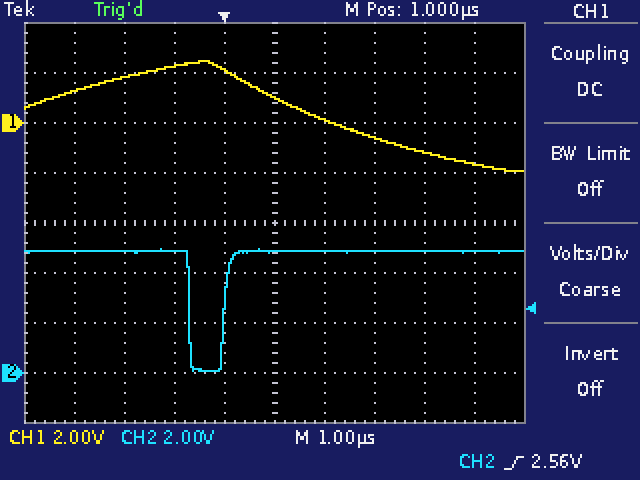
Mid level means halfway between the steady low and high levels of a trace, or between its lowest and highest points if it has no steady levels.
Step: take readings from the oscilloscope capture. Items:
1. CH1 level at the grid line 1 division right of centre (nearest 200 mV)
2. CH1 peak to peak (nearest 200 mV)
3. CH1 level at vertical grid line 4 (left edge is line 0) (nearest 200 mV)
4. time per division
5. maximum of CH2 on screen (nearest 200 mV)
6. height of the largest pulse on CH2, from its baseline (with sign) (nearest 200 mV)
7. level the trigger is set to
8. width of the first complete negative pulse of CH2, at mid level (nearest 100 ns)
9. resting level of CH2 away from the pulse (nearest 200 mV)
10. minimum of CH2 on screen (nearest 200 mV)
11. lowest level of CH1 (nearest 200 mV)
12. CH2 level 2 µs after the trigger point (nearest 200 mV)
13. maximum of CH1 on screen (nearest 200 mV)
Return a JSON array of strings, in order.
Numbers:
["200 mV", "4.4 V", "2.2 V", "1 µs", "5.0 V", "-4.8 V", "2.56 V", "700 ns", "4.8 V", "0.0 V", "-2.0 V", "4.8 V", "2.4 V"]
